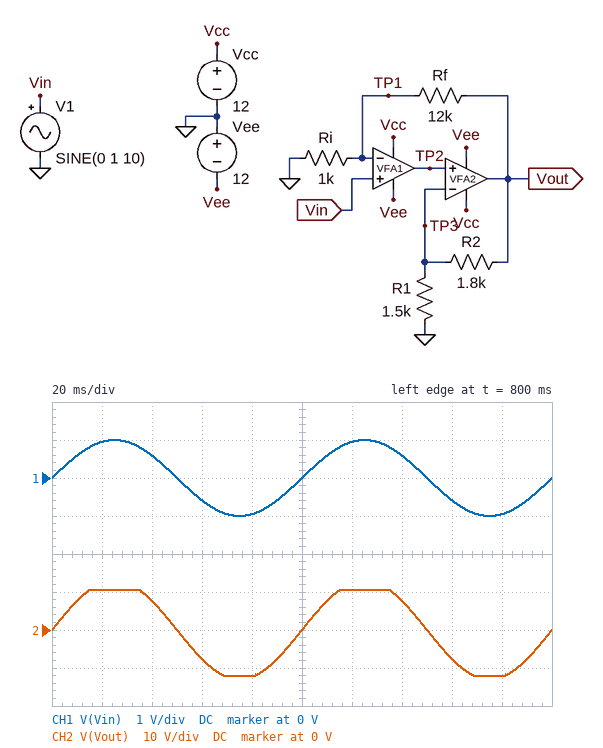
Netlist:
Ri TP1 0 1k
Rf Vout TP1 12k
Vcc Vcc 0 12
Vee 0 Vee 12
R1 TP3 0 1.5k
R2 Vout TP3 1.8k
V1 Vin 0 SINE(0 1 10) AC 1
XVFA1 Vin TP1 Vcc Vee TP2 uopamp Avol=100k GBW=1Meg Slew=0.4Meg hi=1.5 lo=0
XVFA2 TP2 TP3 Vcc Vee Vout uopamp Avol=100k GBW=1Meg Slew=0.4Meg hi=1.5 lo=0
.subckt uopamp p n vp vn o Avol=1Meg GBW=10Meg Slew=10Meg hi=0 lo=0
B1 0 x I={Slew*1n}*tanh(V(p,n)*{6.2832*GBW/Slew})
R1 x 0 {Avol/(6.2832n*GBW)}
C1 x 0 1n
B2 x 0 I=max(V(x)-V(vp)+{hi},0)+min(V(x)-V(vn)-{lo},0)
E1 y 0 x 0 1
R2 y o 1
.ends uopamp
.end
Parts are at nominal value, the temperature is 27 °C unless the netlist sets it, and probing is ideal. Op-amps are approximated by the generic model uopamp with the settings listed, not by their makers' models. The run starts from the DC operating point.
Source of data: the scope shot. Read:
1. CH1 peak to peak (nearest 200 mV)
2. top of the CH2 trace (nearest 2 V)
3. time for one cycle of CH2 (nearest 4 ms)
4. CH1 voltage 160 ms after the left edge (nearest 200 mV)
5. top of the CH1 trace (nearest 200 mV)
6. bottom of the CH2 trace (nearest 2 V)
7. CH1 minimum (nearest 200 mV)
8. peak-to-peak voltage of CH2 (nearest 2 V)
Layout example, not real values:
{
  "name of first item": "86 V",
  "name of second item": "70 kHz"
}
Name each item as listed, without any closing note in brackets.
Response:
{
  "CH1 peak to peak": "2.0 V",
  "top of the CH2 trace": "10 V",
  "time for one cycle of CH2": "100 ms",
  "CH1 voltage 160 ms after the left edge": "-600 mV",
  "top of the CH1 trace": "1.0 V",
  "bottom of the CH2 trace": "-12 V",
  "CH1 minimum": "-1.0 V",
  "peak-to-peak voltage of CH2": "22 V"
}
